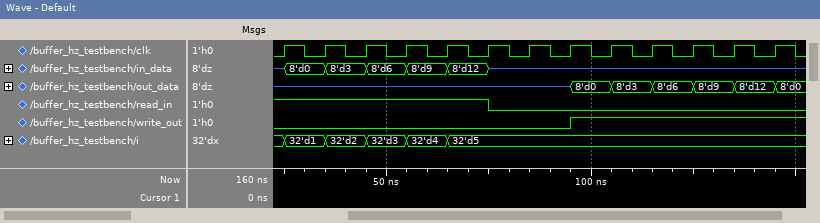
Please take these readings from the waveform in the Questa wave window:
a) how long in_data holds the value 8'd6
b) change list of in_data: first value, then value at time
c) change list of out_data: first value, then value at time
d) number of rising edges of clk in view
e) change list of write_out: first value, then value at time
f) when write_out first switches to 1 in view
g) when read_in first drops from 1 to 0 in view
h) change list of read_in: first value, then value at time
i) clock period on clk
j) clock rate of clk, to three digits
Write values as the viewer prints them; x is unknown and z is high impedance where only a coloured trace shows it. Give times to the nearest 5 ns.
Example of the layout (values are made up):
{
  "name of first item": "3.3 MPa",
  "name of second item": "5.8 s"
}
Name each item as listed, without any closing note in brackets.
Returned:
{
  "how long in_data holds the value 8'd6": "10 ns",
  "change list of in_data: first value, then value at time": "z, 8'd0 at 25 ns, 8'd3 at 35 ns, 8'd6 at 45 ns, 8'd9 at 55 ns, 8'd12 at 65 ns, z at 75 ns",
  "change list of out_data: first value, then value at time": "z, 8'd0 at 95 ns, 8'd3 at 105 ns, 8'd6 at 115 ns, 8'd9 at 125 ns, 8'd12 at 135 ns, 8'd0 at 145 ns",
  "number of rising edges of clk in view": "13",
  "change list of write_out: first value, then value at time": "0, 1 at 95 ns",
  "when write_out first switches to 1 in view": "95 ns",
  "when read_in first drops from 1 to 0 in view": "75 ns",
  "change list of read_in: first value, then value at time": "1, 0 at 75 ns",
  "clock period on clk": "10 ns",
  "clock rate of clk, to three digits": "100 MHz"
}
